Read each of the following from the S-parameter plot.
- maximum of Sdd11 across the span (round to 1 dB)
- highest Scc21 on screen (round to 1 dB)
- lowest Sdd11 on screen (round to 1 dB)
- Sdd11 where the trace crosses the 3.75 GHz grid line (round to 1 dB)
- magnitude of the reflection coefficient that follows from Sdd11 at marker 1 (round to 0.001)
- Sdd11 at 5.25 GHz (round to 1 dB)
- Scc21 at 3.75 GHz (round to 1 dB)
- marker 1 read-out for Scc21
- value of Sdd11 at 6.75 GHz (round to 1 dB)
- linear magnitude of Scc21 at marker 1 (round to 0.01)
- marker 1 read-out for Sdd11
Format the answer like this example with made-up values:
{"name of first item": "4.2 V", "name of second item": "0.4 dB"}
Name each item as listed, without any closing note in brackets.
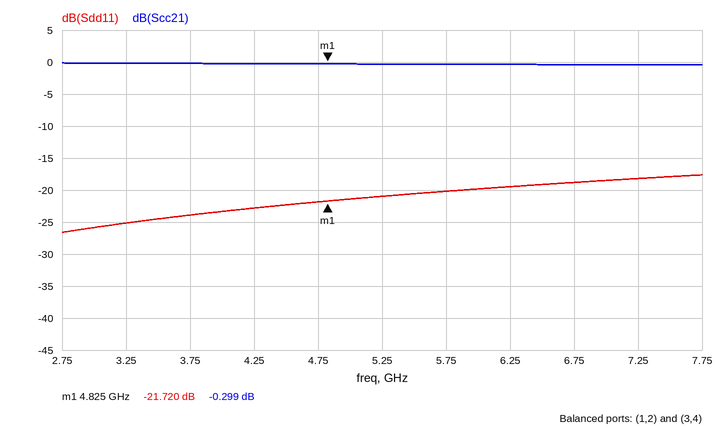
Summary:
{"maximum of Sdd11 across the span": "-18 dB", "highest Scc21 on screen": "0 dB", "lowest Sdd11 on screen": "-27 dB", "Sdd11 where the trace crosses the 3.75 GHz grid line": "-24 dB", "magnitude of the reflection coefficient that follows from Sdd11 at marker 1": "0.082", "Sdd11 at 5.25 GHz": "-21 dB", "Scc21 at 3.75 GHz": "0 dB", "marker 1 read-out for Scc21": "-0.299 dB", "value of Sdd11 at 6.75 GHz": "-19 dB", "linear magnitude of Scc21 at marker 1": "0.97", "marker 1 read-out for Sdd11": "-21.720 dB"}
